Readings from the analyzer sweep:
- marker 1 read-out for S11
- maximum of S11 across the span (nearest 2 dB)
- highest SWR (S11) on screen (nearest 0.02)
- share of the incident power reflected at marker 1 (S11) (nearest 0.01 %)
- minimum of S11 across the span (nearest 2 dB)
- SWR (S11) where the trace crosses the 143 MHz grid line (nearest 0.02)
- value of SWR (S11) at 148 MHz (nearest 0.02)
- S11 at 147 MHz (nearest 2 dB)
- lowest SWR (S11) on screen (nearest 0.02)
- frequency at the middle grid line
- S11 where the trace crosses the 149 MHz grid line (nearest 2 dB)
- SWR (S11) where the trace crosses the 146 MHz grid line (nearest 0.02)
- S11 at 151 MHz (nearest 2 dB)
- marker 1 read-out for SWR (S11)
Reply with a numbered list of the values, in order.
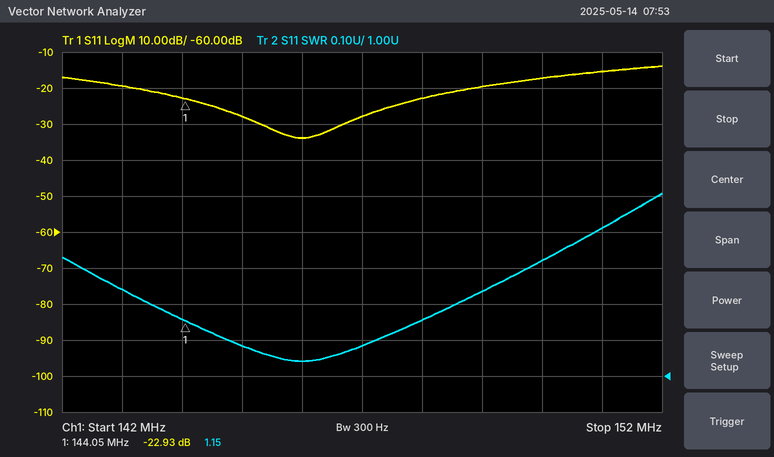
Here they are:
1. -22.93 dB
2. -14 dB
3. 1.50
4. 0.51 %
5. -34 dB
6. 1.24
7. 1.16
8. -28 dB
9. 1.04
10. 147 MHz
11. -20 dB
12. 1.04
13. -16 dB
14. 1.15
